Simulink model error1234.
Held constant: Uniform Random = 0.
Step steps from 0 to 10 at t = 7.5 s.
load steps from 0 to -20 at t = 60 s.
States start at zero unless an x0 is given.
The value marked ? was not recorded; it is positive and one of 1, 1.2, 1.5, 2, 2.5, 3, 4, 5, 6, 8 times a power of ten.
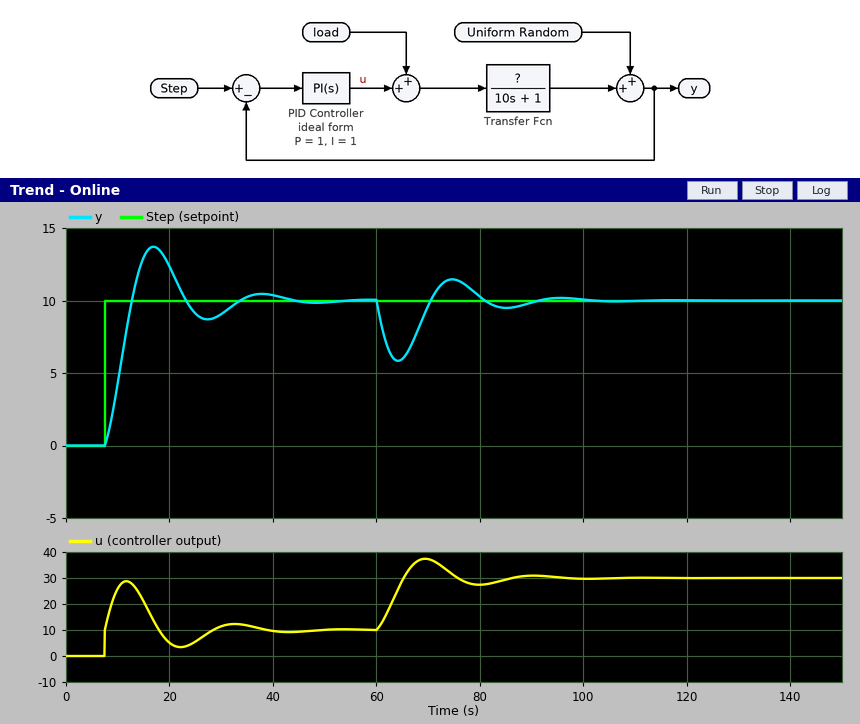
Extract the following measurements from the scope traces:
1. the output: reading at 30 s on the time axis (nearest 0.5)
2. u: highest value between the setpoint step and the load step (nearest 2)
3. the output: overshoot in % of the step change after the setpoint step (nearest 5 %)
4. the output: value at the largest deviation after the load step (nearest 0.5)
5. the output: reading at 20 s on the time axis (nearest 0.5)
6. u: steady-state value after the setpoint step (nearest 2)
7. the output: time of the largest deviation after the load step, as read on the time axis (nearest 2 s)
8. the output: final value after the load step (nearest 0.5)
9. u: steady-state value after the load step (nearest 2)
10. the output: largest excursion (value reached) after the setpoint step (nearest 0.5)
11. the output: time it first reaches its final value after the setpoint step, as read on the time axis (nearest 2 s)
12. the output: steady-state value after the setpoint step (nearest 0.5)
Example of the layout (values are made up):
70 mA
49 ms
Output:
9.0
28
35 %
6.0
12.5
10
64 s
10.0
30
13.5
12 s
10.0
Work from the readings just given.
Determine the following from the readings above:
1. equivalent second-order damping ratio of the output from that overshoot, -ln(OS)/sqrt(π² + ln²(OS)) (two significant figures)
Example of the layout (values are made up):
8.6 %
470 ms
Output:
0.32
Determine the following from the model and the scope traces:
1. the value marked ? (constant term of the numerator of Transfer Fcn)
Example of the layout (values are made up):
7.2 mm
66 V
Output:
1
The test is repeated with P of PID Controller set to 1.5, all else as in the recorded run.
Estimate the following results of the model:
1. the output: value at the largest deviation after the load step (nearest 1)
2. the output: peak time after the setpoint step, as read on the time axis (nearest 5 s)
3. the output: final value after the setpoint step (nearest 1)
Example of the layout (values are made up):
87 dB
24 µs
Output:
7
15 s
10
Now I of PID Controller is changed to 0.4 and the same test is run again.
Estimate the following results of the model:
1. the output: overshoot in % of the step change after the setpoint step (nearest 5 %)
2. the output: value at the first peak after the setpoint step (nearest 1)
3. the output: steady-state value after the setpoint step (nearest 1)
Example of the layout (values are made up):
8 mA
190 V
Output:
20 %
12
10
